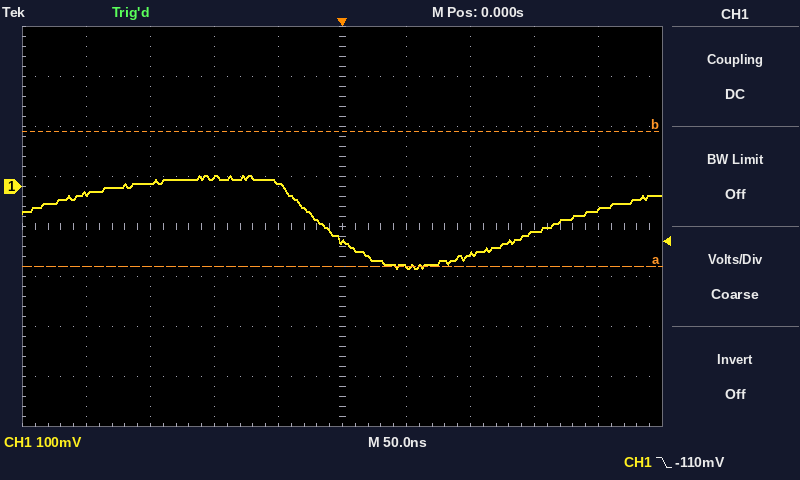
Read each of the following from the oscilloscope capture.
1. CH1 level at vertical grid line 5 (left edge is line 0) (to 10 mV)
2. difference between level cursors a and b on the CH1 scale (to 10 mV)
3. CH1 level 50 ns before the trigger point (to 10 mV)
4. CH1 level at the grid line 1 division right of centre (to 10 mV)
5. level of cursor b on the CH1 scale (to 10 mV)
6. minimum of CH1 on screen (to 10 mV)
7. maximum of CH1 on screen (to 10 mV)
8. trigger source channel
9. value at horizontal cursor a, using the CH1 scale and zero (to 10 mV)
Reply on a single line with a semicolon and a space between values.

-110 mV; 270 mV; 10 mV; -160 mV; 110 mV; -160 mV; 20 mV; CH1; -160 mV
